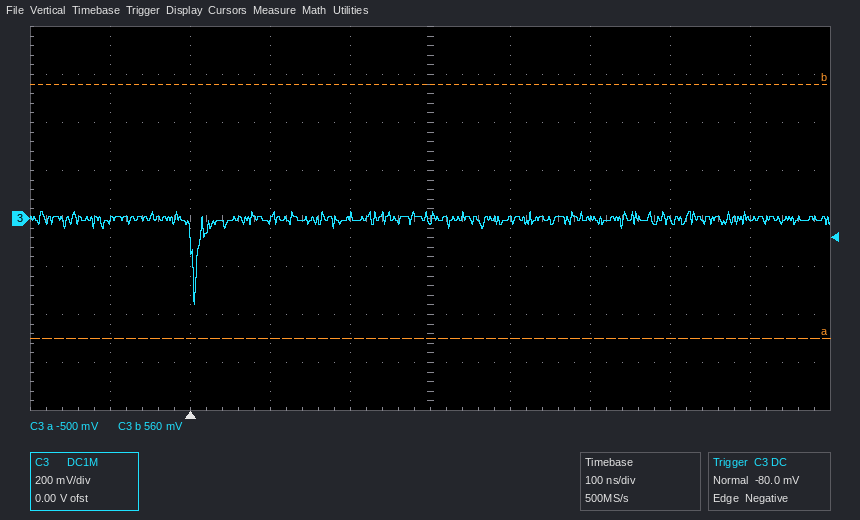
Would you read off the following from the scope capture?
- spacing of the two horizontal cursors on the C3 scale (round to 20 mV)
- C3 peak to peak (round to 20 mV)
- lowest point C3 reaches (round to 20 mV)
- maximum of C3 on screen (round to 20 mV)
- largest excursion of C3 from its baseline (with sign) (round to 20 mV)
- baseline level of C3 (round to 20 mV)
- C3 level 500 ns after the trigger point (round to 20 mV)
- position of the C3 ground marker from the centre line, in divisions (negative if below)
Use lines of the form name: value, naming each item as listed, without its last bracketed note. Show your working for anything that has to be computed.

spacing of the two horizontal cursors on the C3 scale: 1.06 V
C3 peak to peak: 20 mV − (-360 mV) = 380 mV
lowest point C3 reaches: -360 mV
maximum of C3 on screen: 20 mV
largest excursion of C3 from its baseline (with sign): -360 mV − (0 mV) = -360 mV
baseline level of C3: 0 mV
C3 level 500 ns after the trigger point: 0 mV
position of the C3 ground marker from the centre line, in divisions: 0.0 div
